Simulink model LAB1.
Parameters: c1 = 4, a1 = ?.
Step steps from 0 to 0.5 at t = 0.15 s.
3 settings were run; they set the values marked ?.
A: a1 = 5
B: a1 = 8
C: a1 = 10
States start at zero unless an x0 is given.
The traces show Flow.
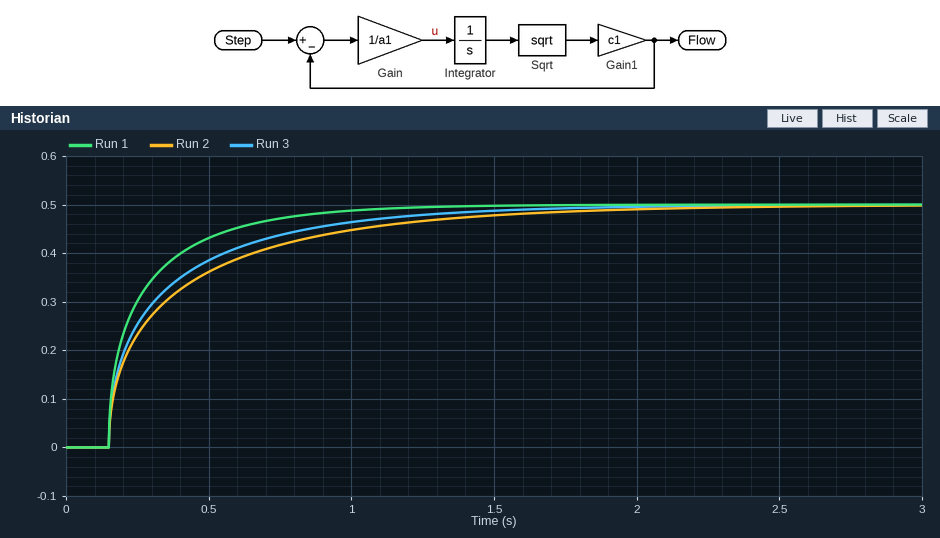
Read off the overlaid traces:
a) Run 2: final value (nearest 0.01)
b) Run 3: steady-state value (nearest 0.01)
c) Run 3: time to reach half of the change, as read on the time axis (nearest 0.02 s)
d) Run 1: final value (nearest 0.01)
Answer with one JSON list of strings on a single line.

["0.50", "0.50", "0.24 s", "0.50"]
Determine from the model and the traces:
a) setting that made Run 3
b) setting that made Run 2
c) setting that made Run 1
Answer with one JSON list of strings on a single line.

["B", "C", "A"]
